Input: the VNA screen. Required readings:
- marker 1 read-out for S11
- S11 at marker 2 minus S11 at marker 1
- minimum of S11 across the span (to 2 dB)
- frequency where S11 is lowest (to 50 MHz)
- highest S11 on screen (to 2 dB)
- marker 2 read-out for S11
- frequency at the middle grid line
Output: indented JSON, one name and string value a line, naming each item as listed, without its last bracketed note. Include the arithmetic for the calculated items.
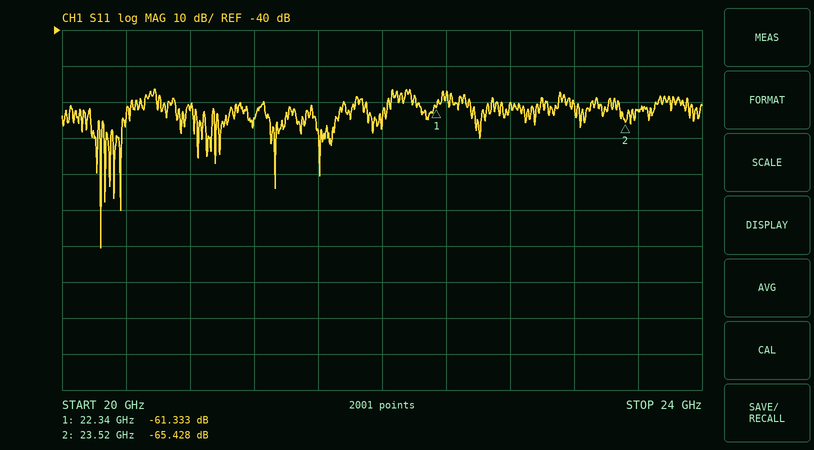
{
  "marker 1 read-out for S11": "-61.333 dB",
  "S11 at marker 2 minus S11 at marker 1": "-65.428 − (-61.333) = -4.095 dB",
  "minimum of S11 across the span": "-100 dB",
  "frequency where S11 is lowest": "20.25 GHz",
  "highest S11 on screen": "-56 dB",
  "marker 2 read-out for S11": "-65.428 dB",
  "frequency at the middle grid line": "22 GHz"
}
